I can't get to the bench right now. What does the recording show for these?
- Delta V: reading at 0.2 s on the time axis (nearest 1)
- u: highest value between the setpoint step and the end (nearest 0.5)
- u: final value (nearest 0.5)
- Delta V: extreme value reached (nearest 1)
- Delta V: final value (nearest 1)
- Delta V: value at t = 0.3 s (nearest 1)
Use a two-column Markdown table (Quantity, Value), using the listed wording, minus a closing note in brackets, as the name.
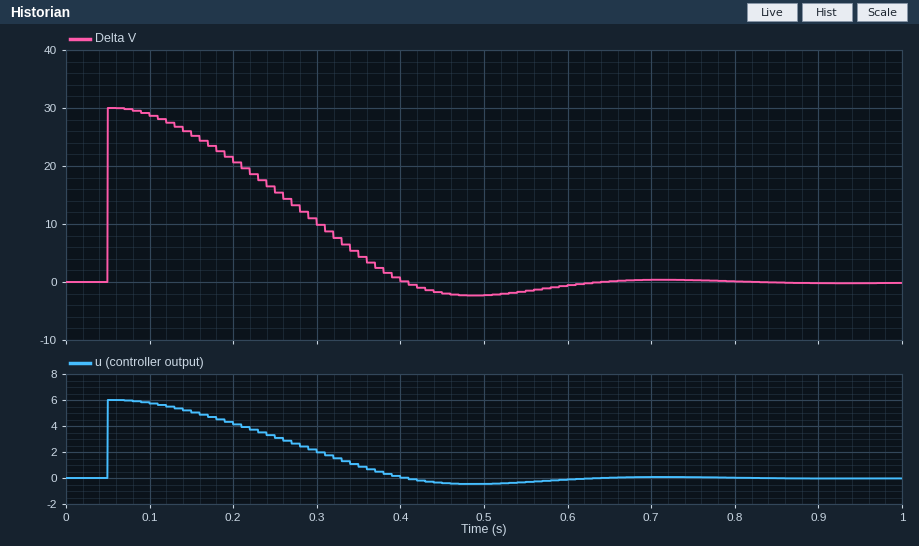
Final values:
| Quantity | Value |
|---|---|
| Delta V: reading at 0.2 s on the time axis | 21 |
| u: highest value between the setpoint step and the end | 6.0 |
| u: final value | 0.0 |
| Delta V: extreme value reached | 30 |
| Delta V: final value | 0 |
| Delta V: value at t = 0.3 s | 10 |
